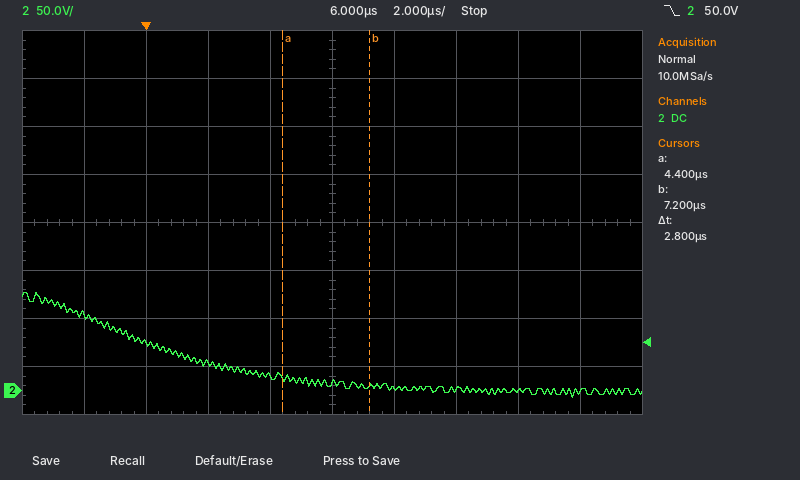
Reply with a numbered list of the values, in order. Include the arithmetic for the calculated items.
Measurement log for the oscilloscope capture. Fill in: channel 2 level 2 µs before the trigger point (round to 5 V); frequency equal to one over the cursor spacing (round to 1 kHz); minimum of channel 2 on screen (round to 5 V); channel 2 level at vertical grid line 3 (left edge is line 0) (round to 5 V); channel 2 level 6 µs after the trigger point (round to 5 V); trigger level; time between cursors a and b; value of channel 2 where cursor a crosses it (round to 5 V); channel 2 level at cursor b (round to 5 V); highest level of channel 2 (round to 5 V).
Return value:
1. 80 V
2. 1 / 2.8 µs ≈ 357 kHz
3. -5 V
4. 30 V
5. 10 V
6. 50.0 V
7. 2.8 µs
8. 15 V
9. 5 V
10. 100 V
